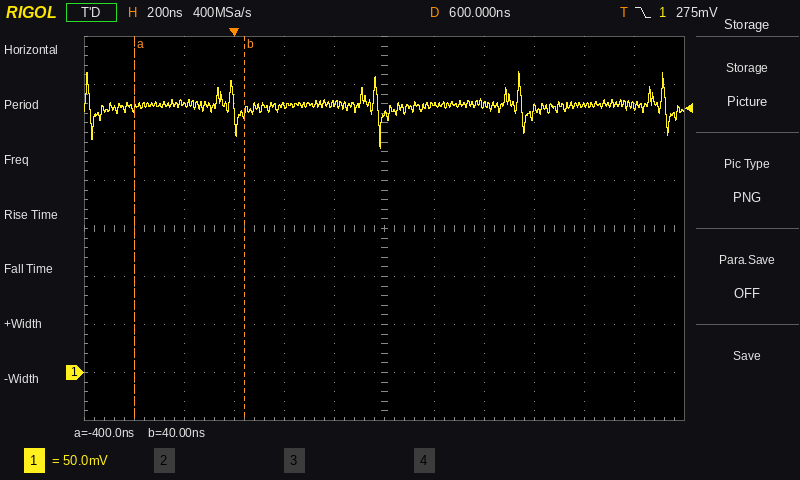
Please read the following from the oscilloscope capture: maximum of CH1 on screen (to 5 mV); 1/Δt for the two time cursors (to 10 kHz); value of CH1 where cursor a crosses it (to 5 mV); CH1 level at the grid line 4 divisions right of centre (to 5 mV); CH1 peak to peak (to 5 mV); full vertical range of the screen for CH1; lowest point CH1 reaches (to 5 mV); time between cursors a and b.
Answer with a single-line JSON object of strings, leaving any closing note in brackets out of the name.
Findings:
{"maximum of CH1 on screen": "315 mV", "1/Δt for the two time cursors": "2.27 MHz", "value of CH1 where cursor a crosses it": "275 mV", "CH1 level at the grid line 4 divisions right of centre": "280 mV", "CH1 peak to peak": "80 mV", "full vertical range of the screen for CH1": "400 mV", "lowest point CH1 reaches": "235 mV", "time between cursors a and b": "440 ns"}
